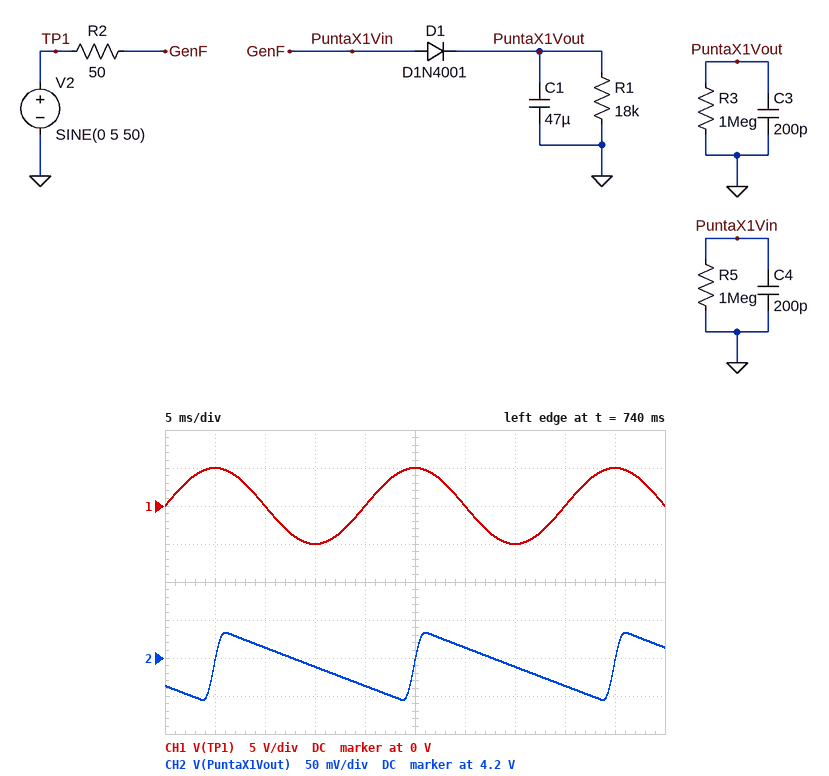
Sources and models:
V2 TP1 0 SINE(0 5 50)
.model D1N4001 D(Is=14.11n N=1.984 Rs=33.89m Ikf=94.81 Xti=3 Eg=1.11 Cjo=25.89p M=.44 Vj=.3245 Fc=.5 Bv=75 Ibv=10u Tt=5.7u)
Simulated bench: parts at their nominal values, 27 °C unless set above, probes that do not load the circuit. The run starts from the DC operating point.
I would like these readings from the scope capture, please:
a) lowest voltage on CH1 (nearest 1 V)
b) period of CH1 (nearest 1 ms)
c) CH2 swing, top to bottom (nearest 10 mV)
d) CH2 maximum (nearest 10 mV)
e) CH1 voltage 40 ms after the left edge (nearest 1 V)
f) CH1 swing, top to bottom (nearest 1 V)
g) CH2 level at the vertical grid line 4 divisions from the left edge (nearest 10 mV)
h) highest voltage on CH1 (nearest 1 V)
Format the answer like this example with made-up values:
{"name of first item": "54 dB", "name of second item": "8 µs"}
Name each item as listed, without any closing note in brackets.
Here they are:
{"lowest voltage on CH1": "-5 V", "period of CH1": "20 ms", "CH2 swing, top to bottom": "90 mV", "CH2 maximum": "4.23 V", "CH1 voltage 40 ms after the left edge": "0 V", "CH1 swing, top to bottom": "10 V", "CH2 level at the vertical grid line 4 divisions from the left edge": "4.16 V", "highest voltage on CH1": "5 V"}
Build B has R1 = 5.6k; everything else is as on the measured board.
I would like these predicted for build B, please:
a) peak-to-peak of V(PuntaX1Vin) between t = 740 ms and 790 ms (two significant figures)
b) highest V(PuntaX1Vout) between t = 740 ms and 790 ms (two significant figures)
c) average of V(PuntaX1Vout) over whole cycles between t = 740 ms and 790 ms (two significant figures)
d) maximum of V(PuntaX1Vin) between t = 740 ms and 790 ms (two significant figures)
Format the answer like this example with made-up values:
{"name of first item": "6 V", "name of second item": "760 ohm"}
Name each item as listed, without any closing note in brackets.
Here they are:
{"peak-to-peak of V(PuntaX1Vin) between t = 740 ms and 790 ms": "9.7 V", "highest V(PuntaX1Vout) between t = 740 ms and 790 ms": "4.1 V", "average of V(PuntaX1Vout) over whole cycles between t = 740 ms and 790 ms": "3.9 V", "maximum of V(PuntaX1Vin) between t = 740 ms and 790 ms": "4.7 V"}
